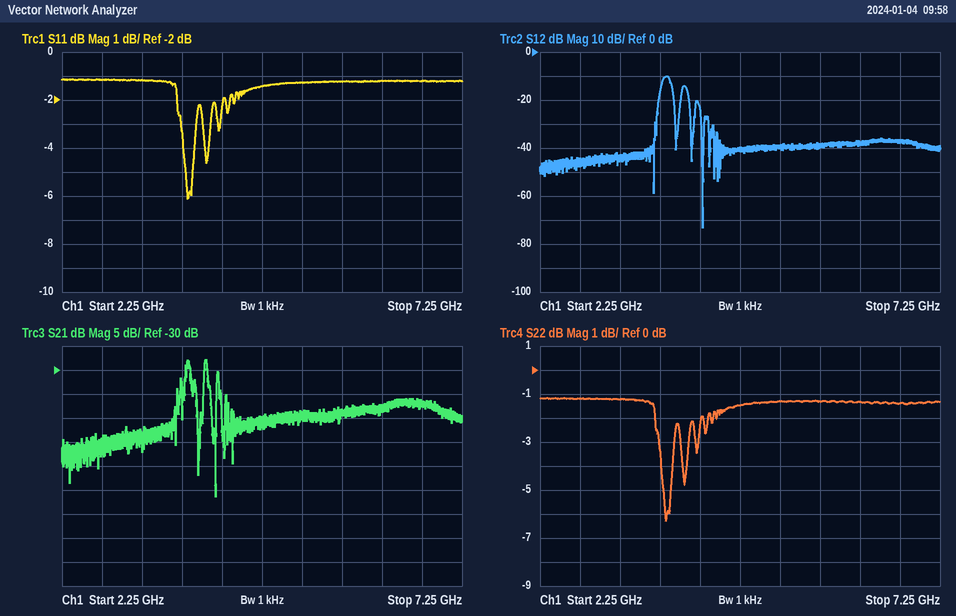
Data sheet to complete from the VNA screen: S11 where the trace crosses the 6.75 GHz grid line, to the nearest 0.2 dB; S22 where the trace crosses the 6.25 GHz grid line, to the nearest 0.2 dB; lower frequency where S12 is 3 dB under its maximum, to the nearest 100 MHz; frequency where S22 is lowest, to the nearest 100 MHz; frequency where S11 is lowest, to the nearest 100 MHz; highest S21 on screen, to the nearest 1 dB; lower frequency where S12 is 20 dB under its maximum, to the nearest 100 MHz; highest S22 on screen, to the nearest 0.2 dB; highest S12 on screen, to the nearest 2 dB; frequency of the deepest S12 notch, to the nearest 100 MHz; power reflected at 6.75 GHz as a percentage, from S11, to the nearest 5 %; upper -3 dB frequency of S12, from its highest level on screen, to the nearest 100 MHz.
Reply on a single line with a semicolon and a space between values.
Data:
-1.2 dB; -1.4 dB; 3.8 GHz; 3.8 GHz; 3.8 GHz; -28 dB; 3.7 GHz; -1.2 dB; -10 dB; 4.3 GHz; 75 %; 3.9 GHz
